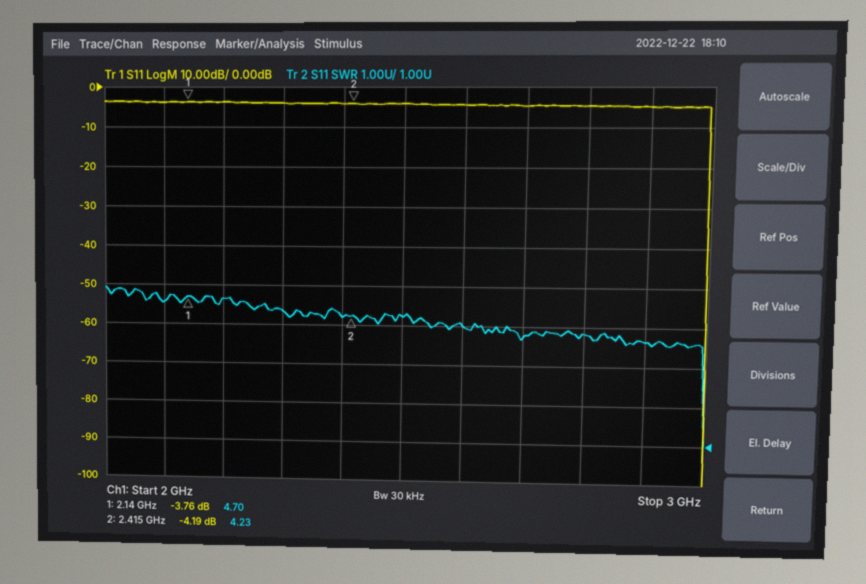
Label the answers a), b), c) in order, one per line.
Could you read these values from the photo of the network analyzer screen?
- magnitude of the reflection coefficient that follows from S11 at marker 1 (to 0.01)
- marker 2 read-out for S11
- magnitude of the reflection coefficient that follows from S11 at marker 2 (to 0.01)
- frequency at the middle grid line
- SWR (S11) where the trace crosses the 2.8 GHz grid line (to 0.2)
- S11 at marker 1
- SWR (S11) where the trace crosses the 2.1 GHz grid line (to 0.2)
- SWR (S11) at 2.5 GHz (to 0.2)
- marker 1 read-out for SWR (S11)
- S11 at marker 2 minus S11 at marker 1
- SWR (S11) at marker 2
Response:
a) 0.65
b) -4.19 dB
c) 0.62
d) 2.5 GHz
e) 3.8
f) -3.76 dB
g) 4.6
h) 4.2
i) 4.70
j) -0.43 dB
k) 4.23
